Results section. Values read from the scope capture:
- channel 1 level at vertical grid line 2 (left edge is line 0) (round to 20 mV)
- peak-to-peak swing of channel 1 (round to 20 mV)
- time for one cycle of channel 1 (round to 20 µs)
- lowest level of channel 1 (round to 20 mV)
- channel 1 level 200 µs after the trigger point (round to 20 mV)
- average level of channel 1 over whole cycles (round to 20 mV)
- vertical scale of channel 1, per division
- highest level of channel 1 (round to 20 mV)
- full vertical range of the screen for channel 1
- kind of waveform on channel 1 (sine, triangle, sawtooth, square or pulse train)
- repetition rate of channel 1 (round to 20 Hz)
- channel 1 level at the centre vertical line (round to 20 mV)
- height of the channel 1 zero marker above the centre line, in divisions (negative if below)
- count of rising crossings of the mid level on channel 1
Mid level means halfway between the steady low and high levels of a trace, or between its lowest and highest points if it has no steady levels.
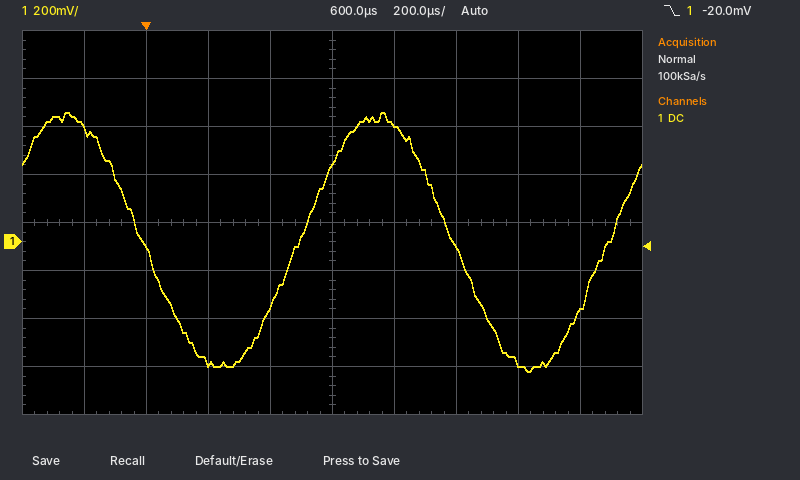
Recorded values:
-20 mV
1.08 V
1.00 ms
-540 mV
-500 mV
0 mV
200 mV
540 mV
1.6 V
sine
1.00 kHz
320 mV
-0.4 div
2
